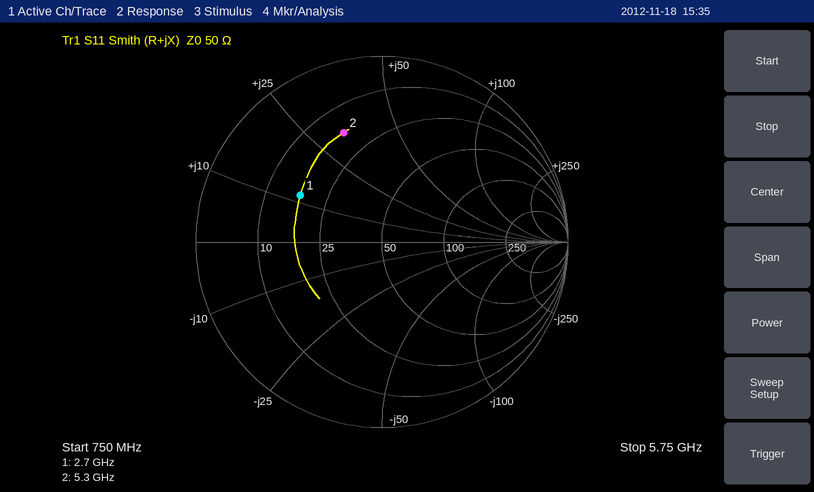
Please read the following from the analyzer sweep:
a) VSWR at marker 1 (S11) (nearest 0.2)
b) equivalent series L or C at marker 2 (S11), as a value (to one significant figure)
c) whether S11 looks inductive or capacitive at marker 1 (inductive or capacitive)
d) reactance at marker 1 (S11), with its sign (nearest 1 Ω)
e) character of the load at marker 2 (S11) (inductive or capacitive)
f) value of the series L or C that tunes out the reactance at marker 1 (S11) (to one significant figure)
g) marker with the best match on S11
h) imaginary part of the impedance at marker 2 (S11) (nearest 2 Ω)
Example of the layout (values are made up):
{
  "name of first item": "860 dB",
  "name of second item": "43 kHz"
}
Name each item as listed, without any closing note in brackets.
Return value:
{
  "VSWR at marker 1 (S11)": "3.0",
  "equivalent series L or C at marker 2 (S11), as a value": "1.0 nH",
  "whether S11 looks inductive or capacitive at marker 1": "inductive",
  "reactance at marker 1 (S11), with its sign": "+12 Ω",
  "character of the load at marker 2 (S11)": "inductive",
  "value of the series L or C that tunes out the reactance at marker 1 (S11)": "5 pF",
  "marker with the best match on S11": "marker 1",
  "imaginary part of the impedance at marker 2 (S11)": "+32 Ω"
}
